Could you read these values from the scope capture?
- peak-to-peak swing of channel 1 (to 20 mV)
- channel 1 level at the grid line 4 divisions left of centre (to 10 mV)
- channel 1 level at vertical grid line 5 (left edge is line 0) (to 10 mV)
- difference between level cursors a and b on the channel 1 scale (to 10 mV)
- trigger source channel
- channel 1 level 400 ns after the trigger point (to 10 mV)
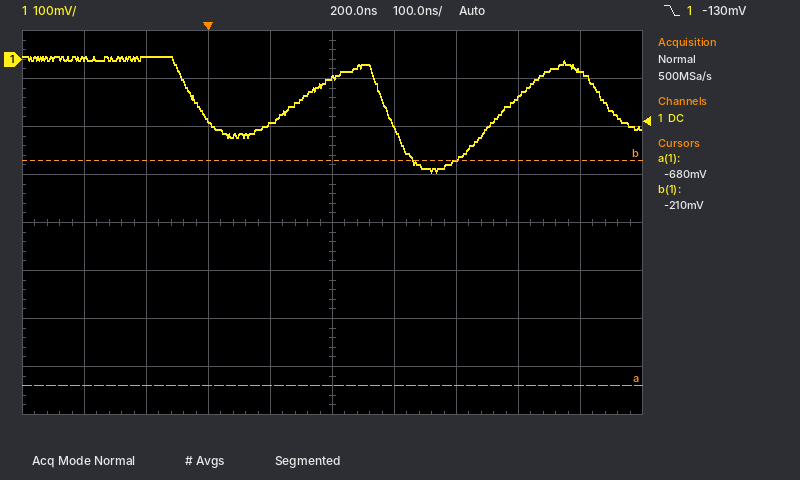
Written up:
240 mV
0 mV
-40 mV
470 mV
channel 1
-210 mV
